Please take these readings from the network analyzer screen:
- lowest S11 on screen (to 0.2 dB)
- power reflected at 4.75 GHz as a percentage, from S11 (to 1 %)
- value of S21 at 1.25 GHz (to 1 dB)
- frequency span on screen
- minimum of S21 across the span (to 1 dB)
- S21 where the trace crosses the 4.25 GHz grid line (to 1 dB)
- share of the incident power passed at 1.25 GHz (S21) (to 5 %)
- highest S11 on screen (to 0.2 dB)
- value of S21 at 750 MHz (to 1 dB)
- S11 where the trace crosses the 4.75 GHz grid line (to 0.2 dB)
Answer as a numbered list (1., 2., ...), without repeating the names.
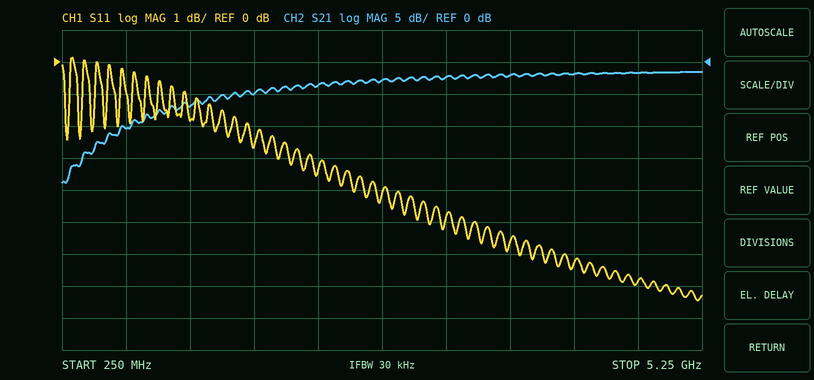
1. -7.4 dB
2. 21 %
3. -7 dB
4. 5 GHz
5. -19 dB
6. -2 dB
7. 20 %
8. 0.2 dB
9. -10 dB
10. -6.8 dB
